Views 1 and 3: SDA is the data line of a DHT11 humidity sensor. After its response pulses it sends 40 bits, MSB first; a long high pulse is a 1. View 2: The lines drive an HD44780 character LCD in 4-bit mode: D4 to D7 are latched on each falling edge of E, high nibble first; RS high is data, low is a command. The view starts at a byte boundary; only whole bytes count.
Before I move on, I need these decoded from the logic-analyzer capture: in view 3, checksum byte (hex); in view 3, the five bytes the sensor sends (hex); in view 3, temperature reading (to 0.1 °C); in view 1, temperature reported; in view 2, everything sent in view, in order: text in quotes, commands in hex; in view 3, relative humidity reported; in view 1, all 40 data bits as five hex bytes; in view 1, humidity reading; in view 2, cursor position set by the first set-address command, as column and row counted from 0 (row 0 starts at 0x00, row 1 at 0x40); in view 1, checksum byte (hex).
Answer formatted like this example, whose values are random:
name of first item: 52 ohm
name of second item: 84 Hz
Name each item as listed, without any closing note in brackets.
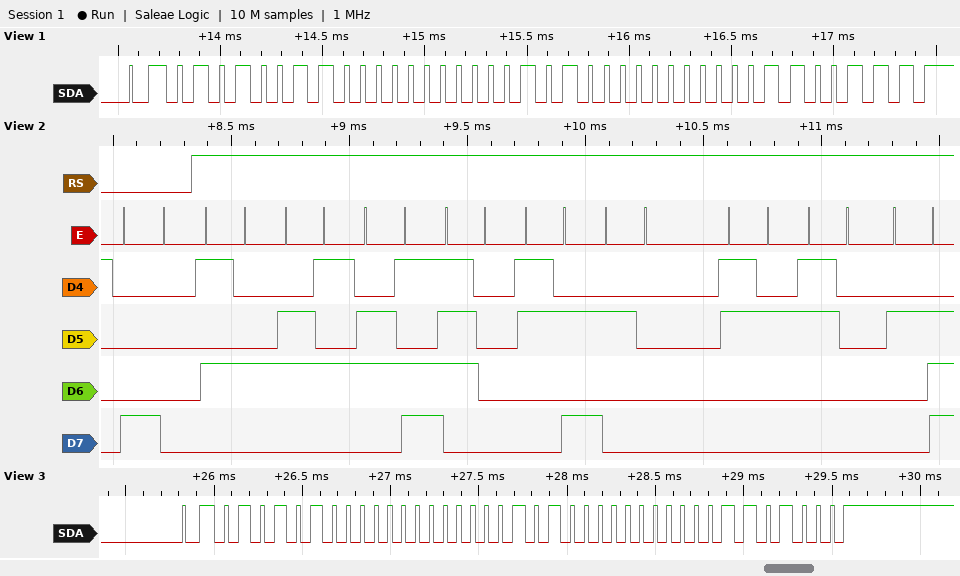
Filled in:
in view 3, checksum byte: 0x68
in view 3, the five bytes the sensor sends: 54 00 14 00 68
in view 3, temperature reading: 20.0 °C
in view 1, temperature reported: 20.0 °C
in view 2, everything sent in view, in order: text in quotes, commands in hex: 0x80 "Temp: 20."
in view 3, relative humidity reported: 84 %
in view 1, all 40 data bits as five hex bytes: 53 00 14 00 67
in view 1, humidity reading: 83 %
in view 2, cursor position set by the first set-address command, as column and row counted from 0: column 0, row 0
in view 1, checksum byte: 0x67
